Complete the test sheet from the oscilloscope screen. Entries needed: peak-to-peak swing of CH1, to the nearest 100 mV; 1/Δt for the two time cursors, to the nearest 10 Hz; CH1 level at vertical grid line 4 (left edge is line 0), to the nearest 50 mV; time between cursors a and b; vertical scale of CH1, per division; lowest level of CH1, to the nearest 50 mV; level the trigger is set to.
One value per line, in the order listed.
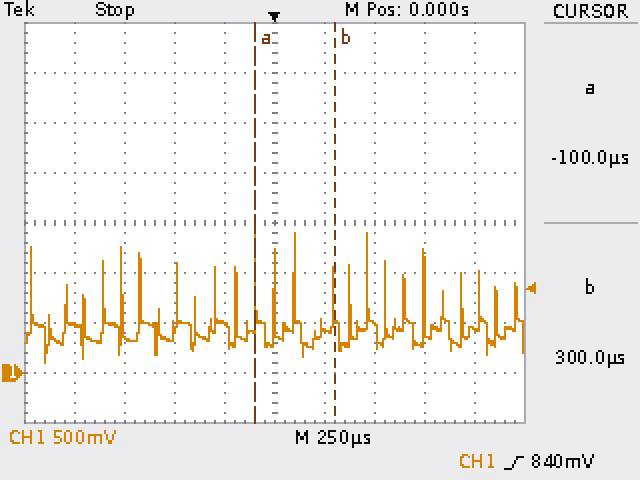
1.30 V
2.50 kHz
500 mV
400 µs
500 mV
100 mV
840 mV
